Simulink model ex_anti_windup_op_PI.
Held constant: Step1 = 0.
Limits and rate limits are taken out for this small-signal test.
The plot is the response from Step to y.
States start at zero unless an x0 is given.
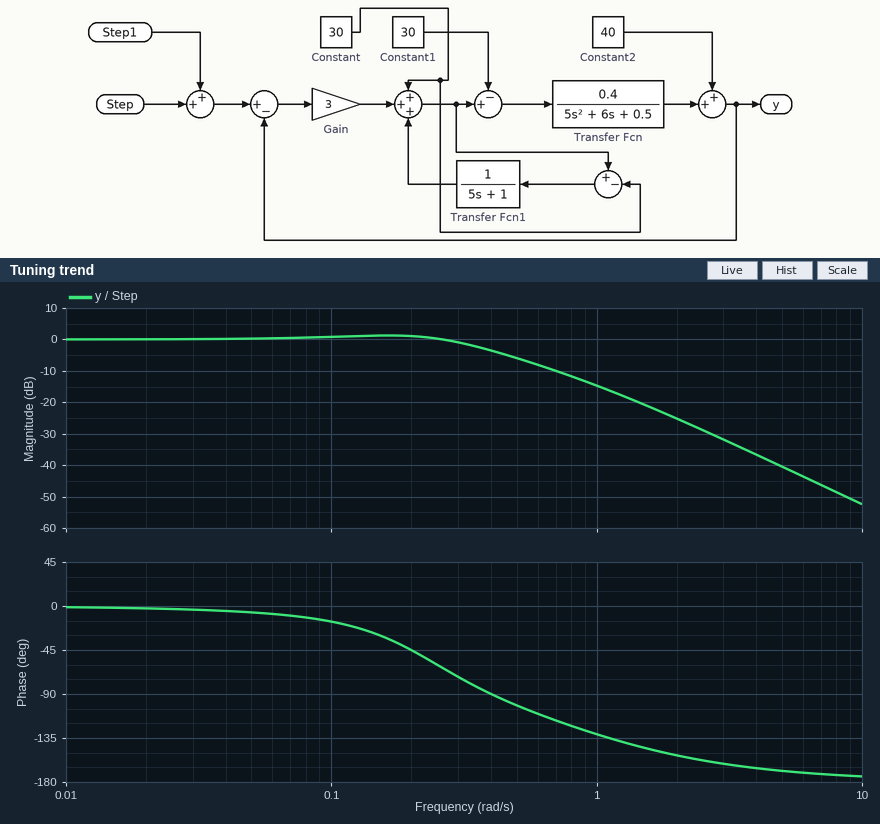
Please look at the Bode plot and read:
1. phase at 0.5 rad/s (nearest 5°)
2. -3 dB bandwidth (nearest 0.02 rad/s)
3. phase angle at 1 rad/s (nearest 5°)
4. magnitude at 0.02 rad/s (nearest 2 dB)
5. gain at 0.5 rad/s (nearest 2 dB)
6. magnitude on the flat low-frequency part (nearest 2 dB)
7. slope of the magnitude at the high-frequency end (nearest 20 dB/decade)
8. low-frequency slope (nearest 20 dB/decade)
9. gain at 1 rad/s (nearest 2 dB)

-100°
0.38 rad/s
-130°
0 dB
-6 dB
0 dB
-40 dB/decade
0 dB/decade
-14 dB
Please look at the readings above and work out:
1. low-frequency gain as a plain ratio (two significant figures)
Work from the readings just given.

1.0
